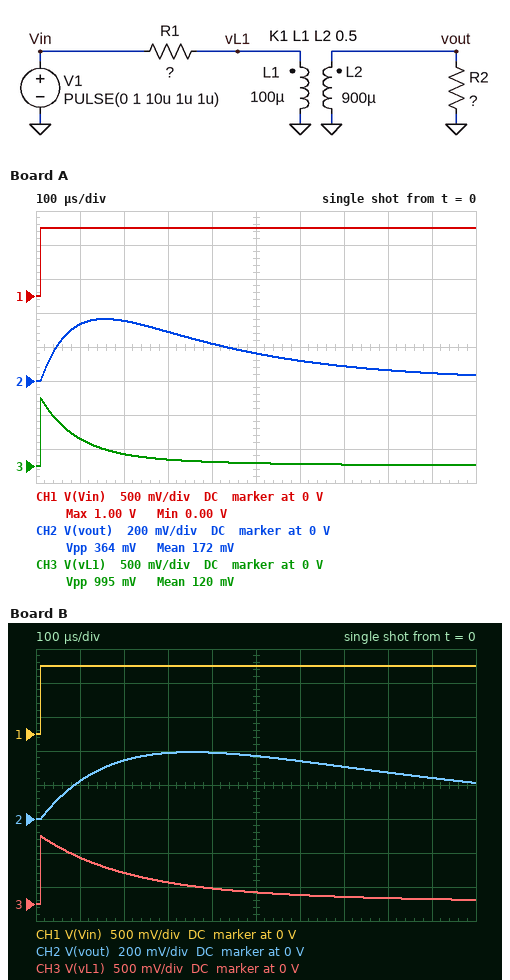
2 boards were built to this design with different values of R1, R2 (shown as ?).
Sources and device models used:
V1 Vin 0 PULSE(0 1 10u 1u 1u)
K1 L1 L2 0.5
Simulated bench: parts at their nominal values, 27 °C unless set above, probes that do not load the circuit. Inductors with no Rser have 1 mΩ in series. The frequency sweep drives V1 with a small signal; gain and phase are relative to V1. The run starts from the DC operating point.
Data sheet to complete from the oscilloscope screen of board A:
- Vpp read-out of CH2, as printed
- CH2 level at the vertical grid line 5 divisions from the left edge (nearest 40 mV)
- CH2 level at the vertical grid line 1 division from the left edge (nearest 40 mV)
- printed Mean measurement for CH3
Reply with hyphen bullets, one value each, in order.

- 364 mV
- 160 mV
- 320 mV
- 120 mV
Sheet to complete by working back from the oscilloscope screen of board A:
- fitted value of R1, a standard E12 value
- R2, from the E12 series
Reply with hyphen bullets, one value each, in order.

- 0.82 Ω
- 3.3 Ω
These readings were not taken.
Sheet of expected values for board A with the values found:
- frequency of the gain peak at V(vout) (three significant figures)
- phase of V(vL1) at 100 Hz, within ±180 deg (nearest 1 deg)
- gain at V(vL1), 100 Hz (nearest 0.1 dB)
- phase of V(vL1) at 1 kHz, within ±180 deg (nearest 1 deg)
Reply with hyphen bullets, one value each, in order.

- 1.01 kHz
- 82 deg
- -22.4 dB
- 52 deg
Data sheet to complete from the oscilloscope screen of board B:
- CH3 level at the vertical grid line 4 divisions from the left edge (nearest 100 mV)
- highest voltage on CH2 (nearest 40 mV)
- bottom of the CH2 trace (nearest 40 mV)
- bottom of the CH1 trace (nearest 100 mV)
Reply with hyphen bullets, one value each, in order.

- 200 mV
- 400 mV
- 0 V
- 0 V
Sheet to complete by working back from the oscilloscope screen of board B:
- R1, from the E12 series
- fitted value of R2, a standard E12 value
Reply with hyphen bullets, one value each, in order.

- 0.33 Ω
- 1.5 Ω
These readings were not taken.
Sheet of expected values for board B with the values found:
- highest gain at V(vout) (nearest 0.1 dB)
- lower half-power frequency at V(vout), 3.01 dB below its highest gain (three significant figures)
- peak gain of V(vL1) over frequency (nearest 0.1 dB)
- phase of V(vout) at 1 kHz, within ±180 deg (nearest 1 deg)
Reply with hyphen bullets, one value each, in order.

- -6.0 dB
- 154 Hz
- 0 dB
- -38 deg
